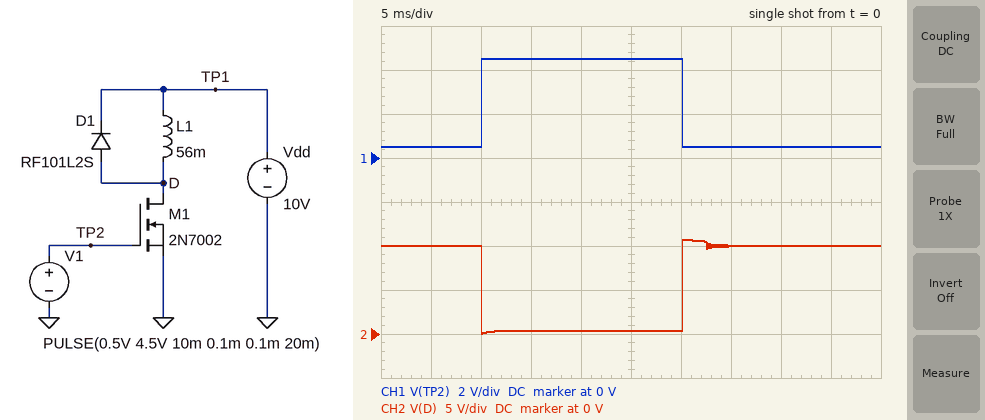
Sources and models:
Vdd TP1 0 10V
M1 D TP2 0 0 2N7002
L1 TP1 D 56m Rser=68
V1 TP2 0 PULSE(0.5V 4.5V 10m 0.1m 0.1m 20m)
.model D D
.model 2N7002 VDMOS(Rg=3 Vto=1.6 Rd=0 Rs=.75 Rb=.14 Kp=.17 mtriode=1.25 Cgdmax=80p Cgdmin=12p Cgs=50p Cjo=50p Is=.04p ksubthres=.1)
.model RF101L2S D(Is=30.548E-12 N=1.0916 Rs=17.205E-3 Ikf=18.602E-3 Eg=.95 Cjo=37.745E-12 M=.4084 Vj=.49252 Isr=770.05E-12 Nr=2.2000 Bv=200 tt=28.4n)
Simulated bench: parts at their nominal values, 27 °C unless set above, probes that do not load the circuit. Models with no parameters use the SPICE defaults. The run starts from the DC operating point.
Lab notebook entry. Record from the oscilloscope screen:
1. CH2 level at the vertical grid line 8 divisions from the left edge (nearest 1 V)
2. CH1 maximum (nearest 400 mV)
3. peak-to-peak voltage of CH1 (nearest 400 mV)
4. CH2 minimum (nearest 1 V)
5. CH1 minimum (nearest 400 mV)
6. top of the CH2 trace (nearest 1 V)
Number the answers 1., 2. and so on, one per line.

1. 10 V
2. 4.4 V
3. 4.0 V
4. 0 V
5. 400 mV
6. 11 V
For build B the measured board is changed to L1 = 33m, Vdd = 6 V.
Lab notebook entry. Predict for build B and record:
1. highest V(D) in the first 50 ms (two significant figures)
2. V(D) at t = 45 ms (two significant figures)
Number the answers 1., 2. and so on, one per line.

1. 6.7 V
2. 6.0 V
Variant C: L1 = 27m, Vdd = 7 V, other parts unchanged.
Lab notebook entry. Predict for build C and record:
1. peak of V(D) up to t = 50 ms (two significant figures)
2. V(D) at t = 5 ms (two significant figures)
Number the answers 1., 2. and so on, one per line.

1. 7.7 V
2. 7.0 V
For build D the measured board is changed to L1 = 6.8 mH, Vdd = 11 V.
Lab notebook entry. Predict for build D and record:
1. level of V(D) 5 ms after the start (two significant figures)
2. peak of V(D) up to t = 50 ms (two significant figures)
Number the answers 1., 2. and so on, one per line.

1. 11 V
2. 12 V
